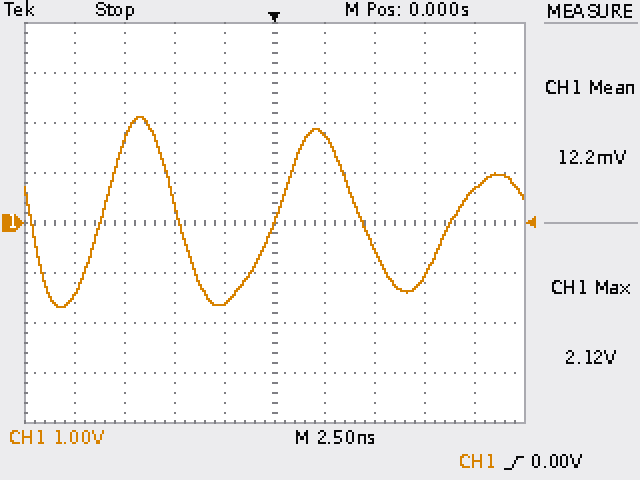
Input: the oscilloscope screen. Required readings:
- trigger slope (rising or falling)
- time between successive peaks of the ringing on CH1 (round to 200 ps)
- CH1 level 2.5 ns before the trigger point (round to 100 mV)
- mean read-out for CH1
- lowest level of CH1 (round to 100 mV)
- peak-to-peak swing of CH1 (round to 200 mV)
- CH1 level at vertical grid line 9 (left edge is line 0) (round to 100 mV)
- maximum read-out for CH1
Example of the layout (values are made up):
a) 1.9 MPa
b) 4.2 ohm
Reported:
a) rising
b) 8.8 ns
c) -1.6 V
d) 12.2 mV
e) -1.7 V
f) 3.8 V
g) 700 mV
h) 2.12 V
